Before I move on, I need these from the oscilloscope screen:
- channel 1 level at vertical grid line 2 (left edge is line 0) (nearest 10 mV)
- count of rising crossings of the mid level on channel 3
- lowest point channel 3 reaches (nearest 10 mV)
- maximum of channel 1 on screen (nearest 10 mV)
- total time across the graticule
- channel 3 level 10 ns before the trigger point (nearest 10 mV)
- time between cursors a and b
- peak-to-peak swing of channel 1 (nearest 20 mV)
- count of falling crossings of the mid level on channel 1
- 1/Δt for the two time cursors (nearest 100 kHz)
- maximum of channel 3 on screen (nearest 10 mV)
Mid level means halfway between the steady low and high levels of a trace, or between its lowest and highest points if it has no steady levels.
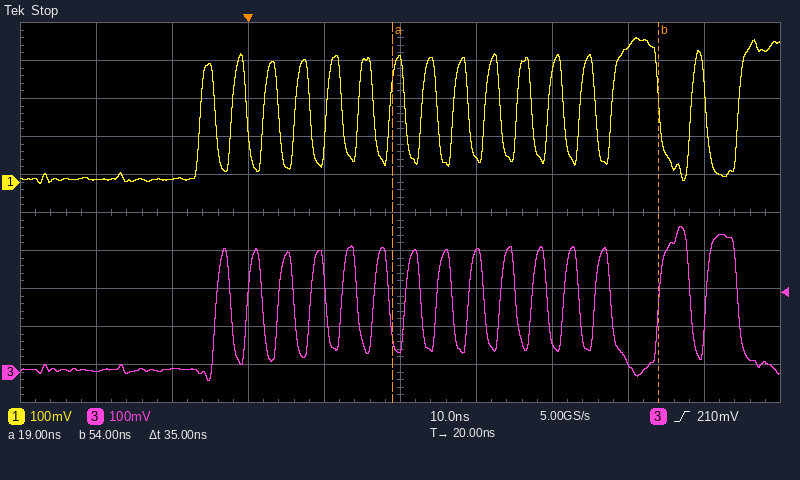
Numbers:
10 mV
15
-20 mV
380 mV
100 ns
10 mV
35 ns
380 mV
15
28.6 MHz
380 mV
